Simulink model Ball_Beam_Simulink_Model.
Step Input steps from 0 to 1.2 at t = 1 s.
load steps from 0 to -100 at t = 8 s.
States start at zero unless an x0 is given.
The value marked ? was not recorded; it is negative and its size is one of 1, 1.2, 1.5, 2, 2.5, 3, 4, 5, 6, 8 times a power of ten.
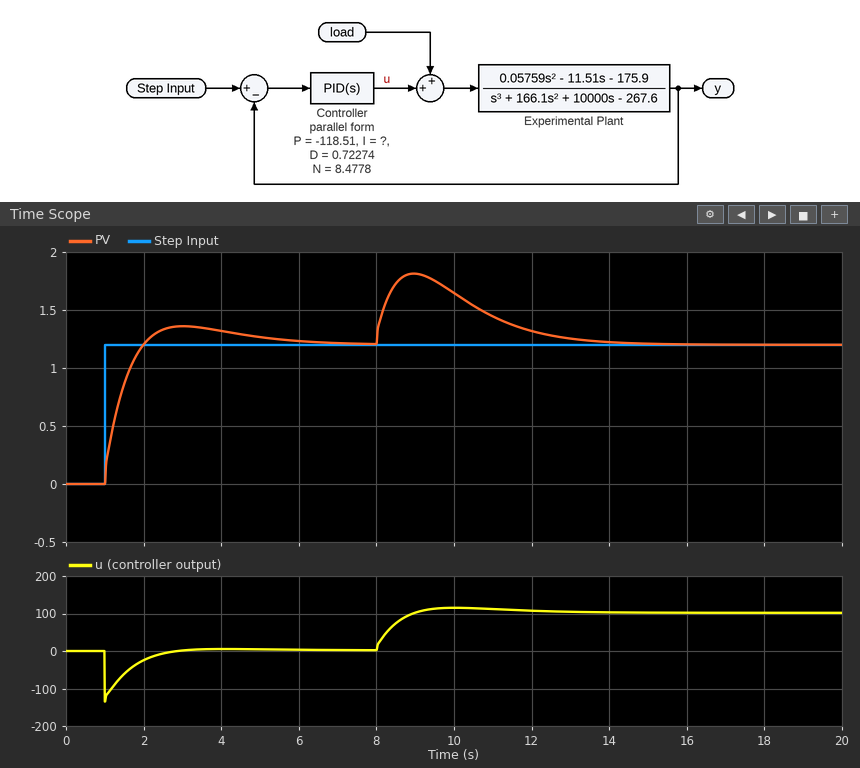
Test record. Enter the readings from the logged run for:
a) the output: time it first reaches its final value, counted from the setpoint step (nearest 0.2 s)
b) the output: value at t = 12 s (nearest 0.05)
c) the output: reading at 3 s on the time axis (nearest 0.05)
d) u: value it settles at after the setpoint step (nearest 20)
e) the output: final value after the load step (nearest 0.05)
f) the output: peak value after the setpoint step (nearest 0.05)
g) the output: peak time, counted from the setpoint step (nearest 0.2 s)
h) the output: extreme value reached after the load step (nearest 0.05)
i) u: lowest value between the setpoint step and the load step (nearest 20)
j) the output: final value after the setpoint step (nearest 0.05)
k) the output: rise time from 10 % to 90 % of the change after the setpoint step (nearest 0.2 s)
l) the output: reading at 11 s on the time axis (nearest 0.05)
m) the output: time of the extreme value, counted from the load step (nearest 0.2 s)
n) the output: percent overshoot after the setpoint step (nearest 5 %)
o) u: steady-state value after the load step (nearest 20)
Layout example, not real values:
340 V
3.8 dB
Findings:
1.0 s
1.30
1.35
0
1.20
1.35
2.0 s
1.80
-140
1.20
0.8 s
1.45
1.0 s
15 %
100
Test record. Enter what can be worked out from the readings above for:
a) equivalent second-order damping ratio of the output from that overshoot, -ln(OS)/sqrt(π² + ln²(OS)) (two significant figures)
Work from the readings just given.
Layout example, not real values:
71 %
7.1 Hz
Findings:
0.52
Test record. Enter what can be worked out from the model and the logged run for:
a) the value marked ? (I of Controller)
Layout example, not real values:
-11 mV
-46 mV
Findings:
-60
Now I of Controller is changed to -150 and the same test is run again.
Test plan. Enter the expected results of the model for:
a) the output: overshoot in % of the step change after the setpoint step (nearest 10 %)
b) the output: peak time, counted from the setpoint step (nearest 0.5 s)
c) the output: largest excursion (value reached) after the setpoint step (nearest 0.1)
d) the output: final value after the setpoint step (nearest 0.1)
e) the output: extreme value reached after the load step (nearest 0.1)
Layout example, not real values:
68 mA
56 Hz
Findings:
20 %
1.5 s
1.5
1.2
1.7
